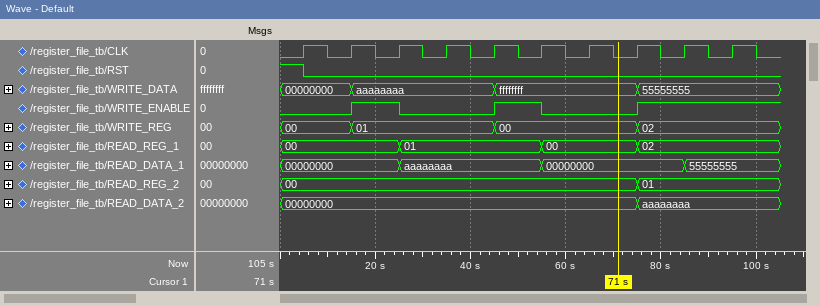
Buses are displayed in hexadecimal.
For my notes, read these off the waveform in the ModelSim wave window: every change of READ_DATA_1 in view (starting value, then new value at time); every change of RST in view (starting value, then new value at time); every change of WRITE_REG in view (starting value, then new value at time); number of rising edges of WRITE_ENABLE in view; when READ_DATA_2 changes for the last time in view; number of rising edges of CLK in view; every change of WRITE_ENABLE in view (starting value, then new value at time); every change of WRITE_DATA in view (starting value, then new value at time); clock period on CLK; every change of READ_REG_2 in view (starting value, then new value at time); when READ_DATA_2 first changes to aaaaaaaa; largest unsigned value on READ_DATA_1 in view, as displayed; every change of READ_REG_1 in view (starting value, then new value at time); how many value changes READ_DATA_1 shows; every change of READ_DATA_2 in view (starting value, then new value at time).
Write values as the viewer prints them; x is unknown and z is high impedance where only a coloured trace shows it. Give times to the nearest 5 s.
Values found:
00000000, aaaaaaaa at 25 s, 00000000 at 55 s, 55555555 at 85 s
1, 0 at 5 s
00, 01 at 15 s, 00 at 45 s, 02 at 75 s
3
75 s
10
0, 1 at 15 s, 0 at 25 s, 1 at 45 s, 0 at 55 s, 1 at 75 s
00000000, aaaaaaaa at 15 s, ffffffff at 45 s, 55555555 at 75 s
10 s
00, 01 at 75 s
75 s
aaaaaaaa
00, 01 at 25 s, 00 at 55 s, 02 at 75 s
3
00000000, aaaaaaaa at 75 s
